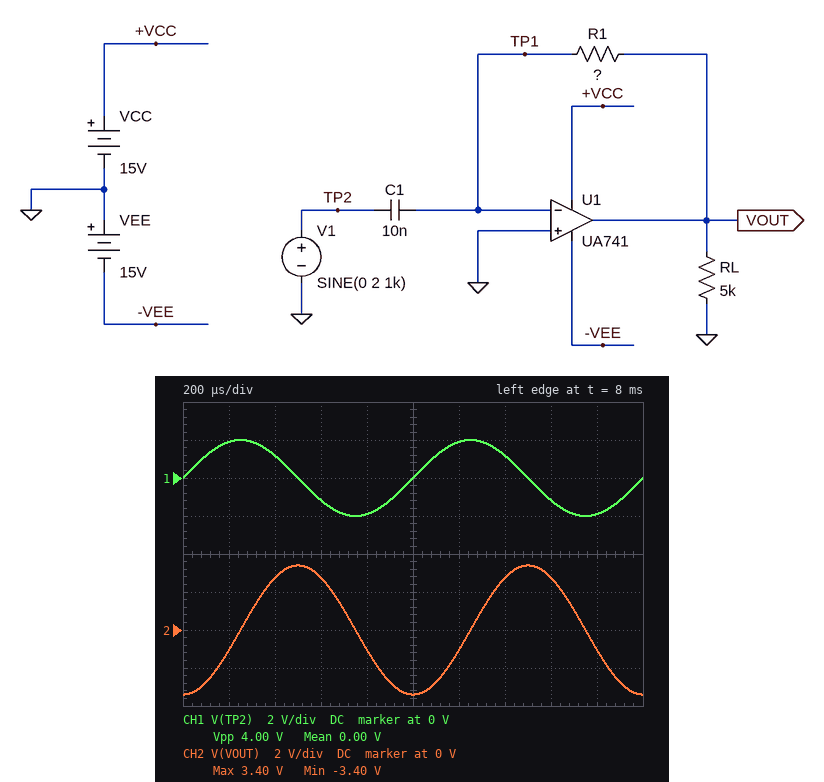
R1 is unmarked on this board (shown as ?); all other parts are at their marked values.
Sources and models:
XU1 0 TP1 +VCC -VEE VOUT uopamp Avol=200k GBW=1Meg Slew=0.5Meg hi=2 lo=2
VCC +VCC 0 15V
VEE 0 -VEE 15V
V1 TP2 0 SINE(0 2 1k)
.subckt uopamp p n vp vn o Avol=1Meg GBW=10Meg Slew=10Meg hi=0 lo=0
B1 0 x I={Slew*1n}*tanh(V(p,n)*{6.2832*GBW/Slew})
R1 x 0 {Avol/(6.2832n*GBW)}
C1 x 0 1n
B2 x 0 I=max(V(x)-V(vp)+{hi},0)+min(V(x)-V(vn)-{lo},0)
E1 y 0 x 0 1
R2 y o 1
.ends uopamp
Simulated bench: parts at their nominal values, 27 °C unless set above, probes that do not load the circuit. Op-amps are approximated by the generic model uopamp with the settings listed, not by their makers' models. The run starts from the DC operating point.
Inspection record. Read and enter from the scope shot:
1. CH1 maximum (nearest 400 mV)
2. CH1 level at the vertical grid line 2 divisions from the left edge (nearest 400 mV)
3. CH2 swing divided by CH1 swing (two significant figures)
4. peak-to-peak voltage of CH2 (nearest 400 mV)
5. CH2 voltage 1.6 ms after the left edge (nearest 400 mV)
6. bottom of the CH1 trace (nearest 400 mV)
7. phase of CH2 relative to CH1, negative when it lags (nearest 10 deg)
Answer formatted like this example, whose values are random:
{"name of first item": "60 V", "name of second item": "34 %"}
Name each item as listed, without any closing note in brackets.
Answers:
{"CH1 maximum": "2.0 V", "CH1 level at the vertical grid line 2 divisions from the left edge": "1.2 V", "CH2 swing divided by CH1 swing": "1.7", "peak-to-peak voltage of CH2": "6.8 V", "CH2 voltage 1.6 ms after the left edge": "2.8 V", "bottom of the CH1 trace": "-2.0 V", "phase of CH2 relative to CH1, negative when it lags": "-90 deg"}
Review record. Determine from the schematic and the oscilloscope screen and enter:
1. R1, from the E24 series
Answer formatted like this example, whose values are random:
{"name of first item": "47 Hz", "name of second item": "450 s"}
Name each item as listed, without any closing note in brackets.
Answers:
{"R1, from the E24 series": "27 kΩ"}
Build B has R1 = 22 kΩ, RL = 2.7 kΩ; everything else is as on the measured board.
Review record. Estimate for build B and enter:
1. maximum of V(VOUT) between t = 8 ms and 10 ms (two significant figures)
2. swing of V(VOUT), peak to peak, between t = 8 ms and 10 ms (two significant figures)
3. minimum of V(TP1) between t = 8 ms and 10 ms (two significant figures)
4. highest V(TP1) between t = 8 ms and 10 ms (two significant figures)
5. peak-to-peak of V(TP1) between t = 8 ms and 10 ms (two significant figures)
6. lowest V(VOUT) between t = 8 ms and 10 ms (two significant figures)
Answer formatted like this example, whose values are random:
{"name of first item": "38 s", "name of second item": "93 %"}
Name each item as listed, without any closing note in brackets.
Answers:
{"maximum of V(VOUT) between t = 8 ms and 10 ms": "2.8 V", "swing of V(VOUT), peak to peak, between t = 8 ms and 10 ms": "5.5 V", "minimum of V(TP1) between t = 8 ms and 10 ms": "-2.8 mV", "highest V(TP1) between t = 8 ms and 10 ms": "2.8 mV", "peak-to-peak of V(TP1) between t = 8 ms and 10 ms": "5.5 mV", "lowest V(VOUT) between t = 8 ms and 10 ms": "-2.8 V"}
